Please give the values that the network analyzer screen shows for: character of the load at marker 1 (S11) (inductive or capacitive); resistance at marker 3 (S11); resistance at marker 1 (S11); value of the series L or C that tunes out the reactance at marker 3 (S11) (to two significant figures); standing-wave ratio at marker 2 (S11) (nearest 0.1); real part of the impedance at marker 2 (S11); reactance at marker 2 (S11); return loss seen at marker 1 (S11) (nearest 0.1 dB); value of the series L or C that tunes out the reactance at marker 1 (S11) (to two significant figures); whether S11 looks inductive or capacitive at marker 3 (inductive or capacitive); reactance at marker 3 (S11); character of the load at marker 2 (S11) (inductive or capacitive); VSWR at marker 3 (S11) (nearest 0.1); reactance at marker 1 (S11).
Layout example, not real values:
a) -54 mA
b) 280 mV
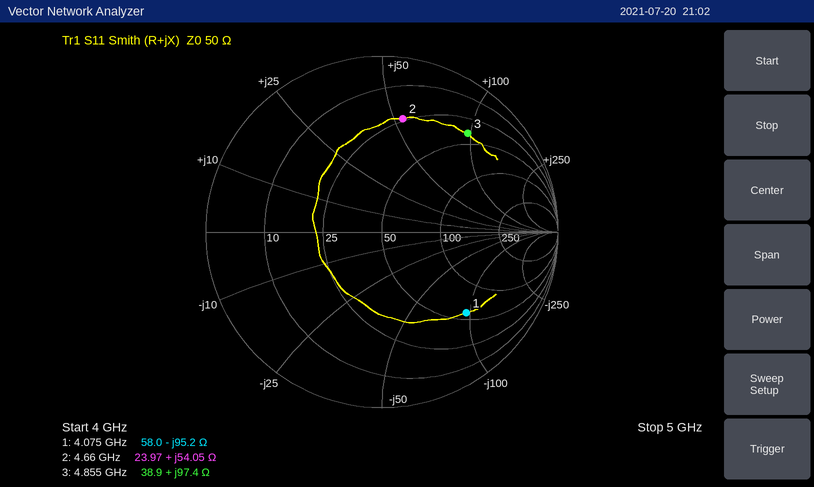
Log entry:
a) capacitive
b) 38.9 Ω
c) 58.0 Ω
d) 340 fF
e) 4.8
f) 23.97 Ω
g) +54.05 Ω
h) 3.6 dB
i) 3.7 nH
j) inductive
k) +97.4 Ω
l) inductive
m) 6.8
n) -95.2 Ω
